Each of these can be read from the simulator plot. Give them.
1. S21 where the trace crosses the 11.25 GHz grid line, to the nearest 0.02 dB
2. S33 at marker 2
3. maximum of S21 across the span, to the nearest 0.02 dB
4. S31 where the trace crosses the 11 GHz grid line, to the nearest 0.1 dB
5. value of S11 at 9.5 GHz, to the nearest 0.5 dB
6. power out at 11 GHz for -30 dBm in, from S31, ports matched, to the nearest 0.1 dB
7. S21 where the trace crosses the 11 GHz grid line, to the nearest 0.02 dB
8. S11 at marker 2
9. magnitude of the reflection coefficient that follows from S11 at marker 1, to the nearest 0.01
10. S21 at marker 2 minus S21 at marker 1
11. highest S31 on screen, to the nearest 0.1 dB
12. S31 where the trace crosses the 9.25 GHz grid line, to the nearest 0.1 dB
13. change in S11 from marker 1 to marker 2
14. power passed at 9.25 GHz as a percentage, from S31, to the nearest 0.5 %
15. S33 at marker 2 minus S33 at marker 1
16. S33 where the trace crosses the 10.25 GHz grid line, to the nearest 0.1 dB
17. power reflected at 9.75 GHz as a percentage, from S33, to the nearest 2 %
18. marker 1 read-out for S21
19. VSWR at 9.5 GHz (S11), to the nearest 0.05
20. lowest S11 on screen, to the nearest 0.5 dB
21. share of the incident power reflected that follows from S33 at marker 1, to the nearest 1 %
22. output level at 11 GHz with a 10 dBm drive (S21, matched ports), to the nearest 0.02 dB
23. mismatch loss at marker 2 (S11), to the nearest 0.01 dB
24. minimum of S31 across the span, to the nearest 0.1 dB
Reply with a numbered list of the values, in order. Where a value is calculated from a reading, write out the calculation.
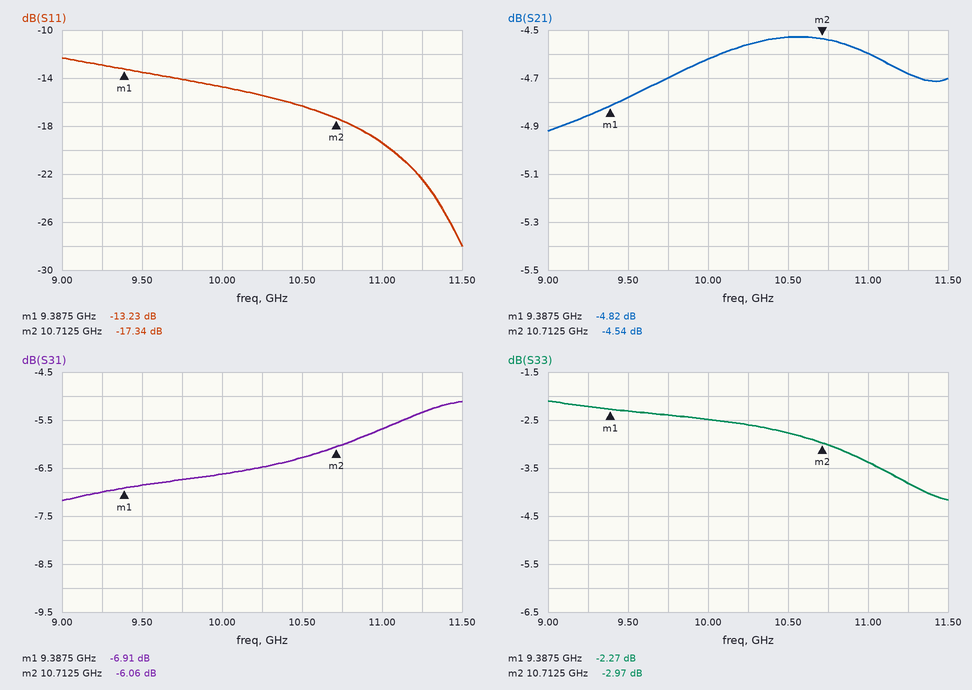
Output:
1. -4.68 dB
2. -2.97 dB
3. -4.52 dB
4. -5.7 dB
5. -13.5 dB
6. -30 dBm + (-5.7 dB) = -35.7 dBm
7. -4.60 dB
8. -17.34 dB
9. 10^(-13.23/20) ≈ 0.22
10. -4.54 − (-4.82) = 0.28 dB
11. -5.1 dB
12. -7.0 dB
13. -17.34 − (-13.23) = -4.11 dB
14. 10^(-7/10) ≈ 20.0 %
15. -2.97 − (-2.27) = -0.70 dB
16. -2.6 dB
17. 10^(-2.4/10) ≈ 58 %
18. -4.82 dB
19. |Γ| = 10^(-13.5/20) = 0.2113; VSWR = (1 + 0.2113)/(1 − 0.2113) ≈ 1.54, so 1.55 to the nearest 0.05
20. -28.0 dB
21. 10^(-2.27/10) ≈ 59 %
22. 10 dBm + (-4.60 dB) = 5.40 dBm
23. −10 log10(1 − 10^(-17.34/10)) ≈ 0.08 dB
24. -7.2 dB
